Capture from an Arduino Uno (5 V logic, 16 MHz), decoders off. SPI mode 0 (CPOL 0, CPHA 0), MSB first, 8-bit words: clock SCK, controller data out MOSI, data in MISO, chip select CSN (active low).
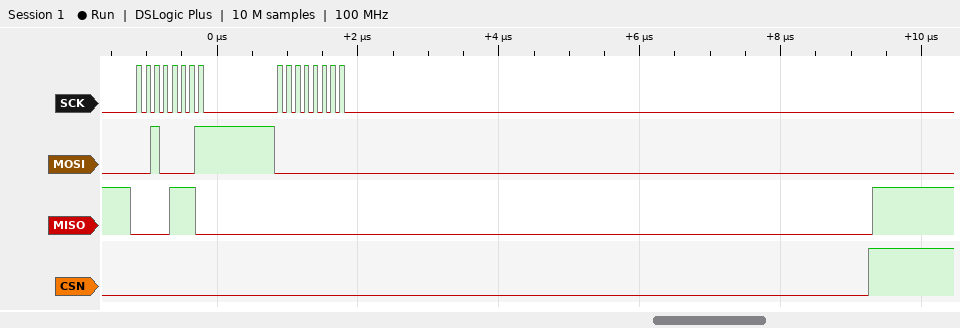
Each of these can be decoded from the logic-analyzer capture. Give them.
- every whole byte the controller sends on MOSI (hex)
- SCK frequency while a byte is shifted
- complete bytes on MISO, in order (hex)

21 00
8 MHz
0E 00
